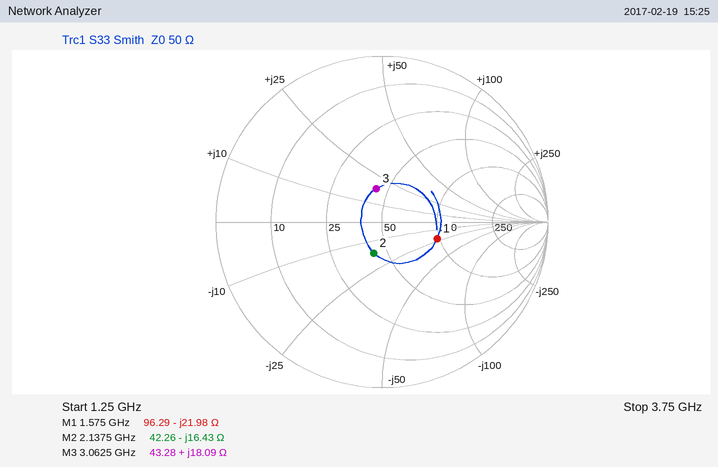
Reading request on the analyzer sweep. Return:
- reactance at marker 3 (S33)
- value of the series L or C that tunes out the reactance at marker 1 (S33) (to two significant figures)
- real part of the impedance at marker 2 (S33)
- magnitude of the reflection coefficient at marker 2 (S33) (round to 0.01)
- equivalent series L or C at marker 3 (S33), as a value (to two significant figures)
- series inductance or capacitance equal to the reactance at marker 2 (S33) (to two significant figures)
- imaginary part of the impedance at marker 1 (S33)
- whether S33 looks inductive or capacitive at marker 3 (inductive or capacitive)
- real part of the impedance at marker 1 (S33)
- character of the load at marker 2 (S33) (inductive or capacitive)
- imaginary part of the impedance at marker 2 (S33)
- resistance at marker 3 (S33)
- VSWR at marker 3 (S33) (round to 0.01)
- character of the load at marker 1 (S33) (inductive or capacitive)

+18.09 Ω
2.2 nH
42.26 Ω
0.19
940 pH
4.5 pF
-21.98 Ω
inductive
96.29 Ω
capacitive
-16.43 Ω
43.28 Ω
1.51
capacitive
